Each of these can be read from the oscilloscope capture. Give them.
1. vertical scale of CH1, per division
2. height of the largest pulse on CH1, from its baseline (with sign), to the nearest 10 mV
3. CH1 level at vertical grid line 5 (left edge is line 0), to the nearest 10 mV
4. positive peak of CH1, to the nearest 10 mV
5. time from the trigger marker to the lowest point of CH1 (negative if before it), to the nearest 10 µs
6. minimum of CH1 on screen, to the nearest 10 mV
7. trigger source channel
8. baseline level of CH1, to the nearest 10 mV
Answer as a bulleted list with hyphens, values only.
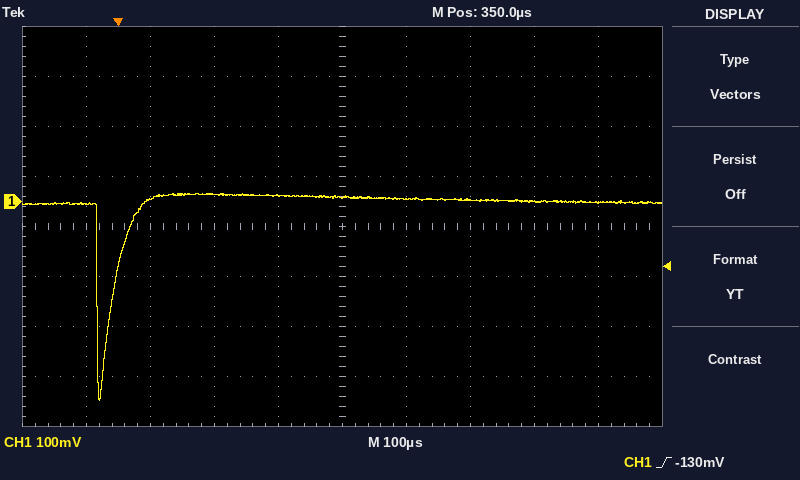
- 100 mV
- -400 mV
- 10 mV
- 20 mV
- -30 µs
- -400 mV
- CH1
- 0 mV
